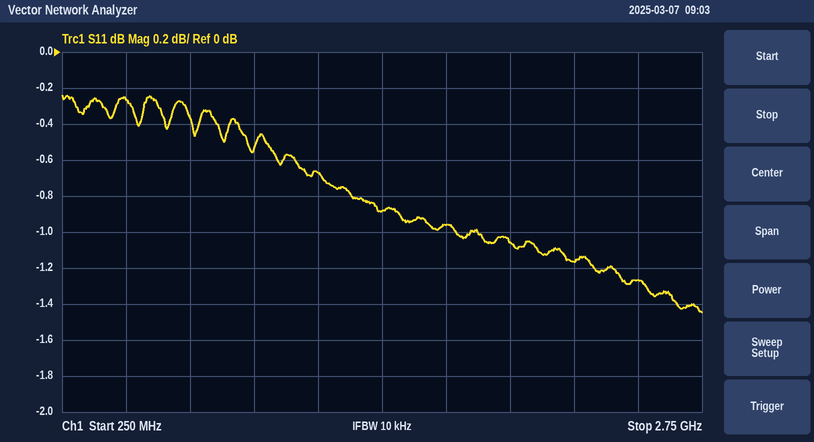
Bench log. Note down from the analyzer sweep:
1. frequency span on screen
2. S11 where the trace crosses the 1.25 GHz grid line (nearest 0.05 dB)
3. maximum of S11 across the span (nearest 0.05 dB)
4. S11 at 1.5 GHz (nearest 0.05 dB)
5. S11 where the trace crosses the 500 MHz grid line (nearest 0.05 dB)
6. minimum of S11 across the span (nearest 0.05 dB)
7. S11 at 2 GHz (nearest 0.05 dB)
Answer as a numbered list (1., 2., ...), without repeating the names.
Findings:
1. 2.5 GHz
2. -0.65 dB
3. -0.25 dB
4. -0.90 dB
5. -0.25 dB
6. -1.45 dB
7. -1.05 dB
